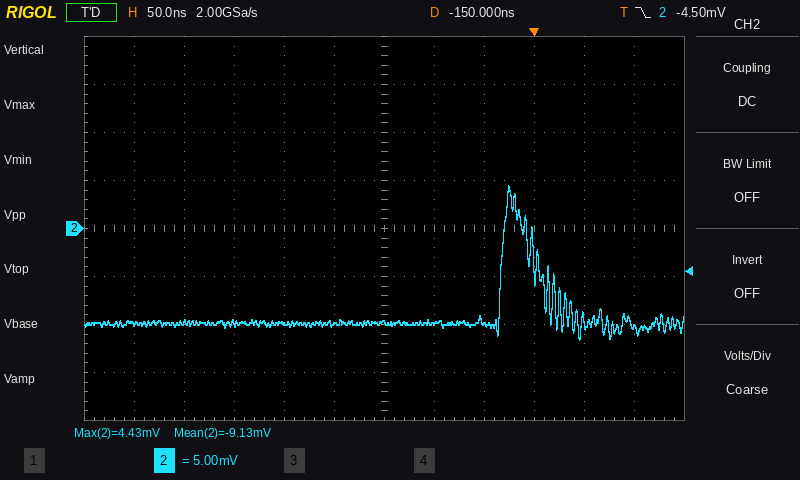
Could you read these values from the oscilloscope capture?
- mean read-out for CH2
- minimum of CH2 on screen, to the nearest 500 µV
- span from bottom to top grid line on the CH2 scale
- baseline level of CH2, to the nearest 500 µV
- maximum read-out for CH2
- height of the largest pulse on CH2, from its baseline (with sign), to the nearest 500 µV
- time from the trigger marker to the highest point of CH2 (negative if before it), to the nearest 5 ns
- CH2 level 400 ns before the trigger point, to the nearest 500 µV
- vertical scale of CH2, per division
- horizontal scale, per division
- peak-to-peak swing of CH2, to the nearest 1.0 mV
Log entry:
-9.13 mV
-11.5 mV
40 mV
-10.0 mV
4.43 mV
+14.5 mV
-25 ns
-10.0 mV
5 mV
50 ns
16.0 mV
